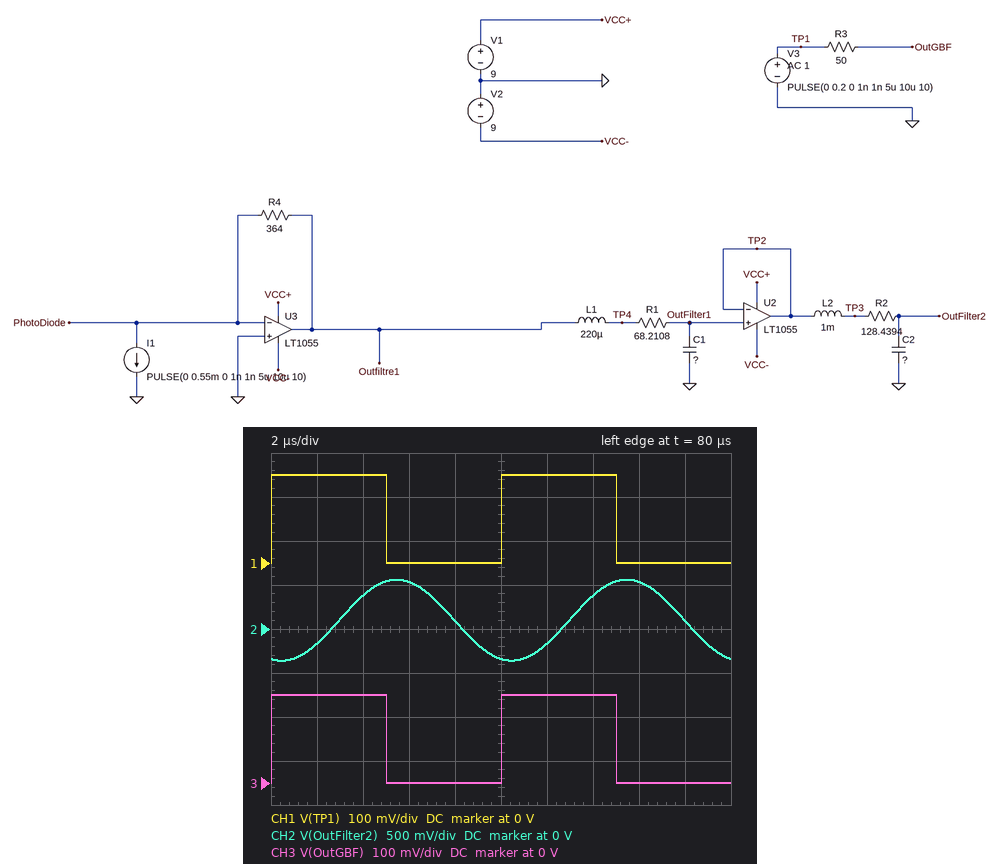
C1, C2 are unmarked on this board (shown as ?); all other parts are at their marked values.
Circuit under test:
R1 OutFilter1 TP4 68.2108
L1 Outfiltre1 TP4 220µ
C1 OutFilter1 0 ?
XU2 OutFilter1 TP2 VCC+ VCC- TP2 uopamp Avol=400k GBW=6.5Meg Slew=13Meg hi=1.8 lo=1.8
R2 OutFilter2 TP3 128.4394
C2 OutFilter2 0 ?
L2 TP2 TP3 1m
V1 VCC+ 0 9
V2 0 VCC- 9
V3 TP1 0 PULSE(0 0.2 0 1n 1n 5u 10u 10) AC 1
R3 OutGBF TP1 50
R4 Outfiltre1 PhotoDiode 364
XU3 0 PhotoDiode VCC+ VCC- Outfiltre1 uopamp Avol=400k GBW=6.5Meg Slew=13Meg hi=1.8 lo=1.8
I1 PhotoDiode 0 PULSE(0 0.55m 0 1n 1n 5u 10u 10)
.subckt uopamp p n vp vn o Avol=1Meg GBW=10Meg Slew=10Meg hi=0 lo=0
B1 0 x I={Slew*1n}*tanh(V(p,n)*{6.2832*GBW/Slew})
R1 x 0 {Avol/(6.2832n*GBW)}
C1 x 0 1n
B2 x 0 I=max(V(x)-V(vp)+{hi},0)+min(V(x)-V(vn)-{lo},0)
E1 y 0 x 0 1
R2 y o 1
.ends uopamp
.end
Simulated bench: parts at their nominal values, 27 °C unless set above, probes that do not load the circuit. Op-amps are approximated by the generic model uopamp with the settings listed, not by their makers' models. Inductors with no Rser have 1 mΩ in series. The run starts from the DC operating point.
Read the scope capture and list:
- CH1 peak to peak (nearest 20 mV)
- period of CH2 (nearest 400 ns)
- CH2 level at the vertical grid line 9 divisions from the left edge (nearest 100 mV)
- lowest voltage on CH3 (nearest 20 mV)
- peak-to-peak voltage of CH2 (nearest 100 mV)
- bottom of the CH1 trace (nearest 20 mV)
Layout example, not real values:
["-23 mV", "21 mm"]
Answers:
["200 mV", "10.0 µs", "100 mV", "0 V", "900 mV", "0 V"]
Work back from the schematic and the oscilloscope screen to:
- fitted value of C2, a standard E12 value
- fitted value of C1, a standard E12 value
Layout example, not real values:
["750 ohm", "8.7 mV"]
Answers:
["1.2 nF", "12 nF"]
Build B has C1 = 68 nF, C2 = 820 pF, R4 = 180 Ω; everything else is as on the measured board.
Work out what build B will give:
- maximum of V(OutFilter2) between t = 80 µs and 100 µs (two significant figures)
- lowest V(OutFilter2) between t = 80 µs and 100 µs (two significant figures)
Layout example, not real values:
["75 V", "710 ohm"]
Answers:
["66 mV", "33 mV"]
